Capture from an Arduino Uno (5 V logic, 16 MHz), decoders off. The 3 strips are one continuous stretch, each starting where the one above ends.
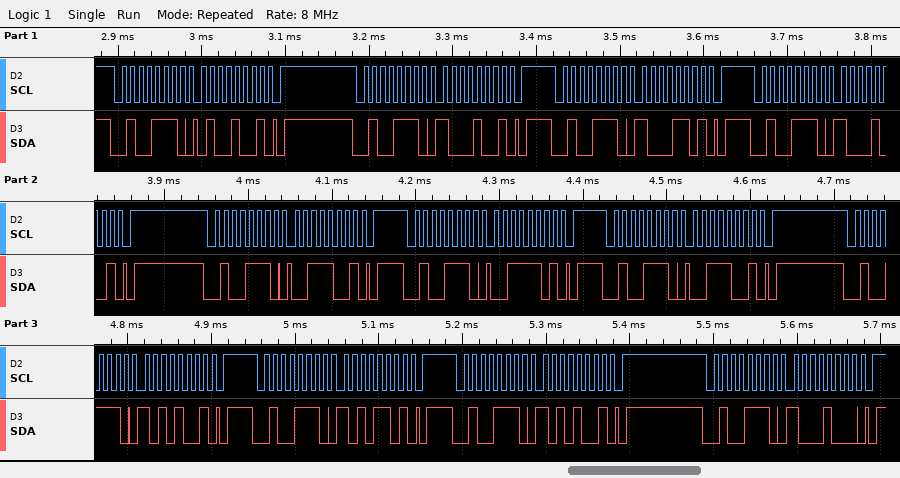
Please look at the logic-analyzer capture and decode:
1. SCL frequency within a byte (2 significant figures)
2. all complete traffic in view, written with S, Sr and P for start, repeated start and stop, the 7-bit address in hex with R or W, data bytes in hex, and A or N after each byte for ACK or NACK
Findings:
100 kHz
S 27W A 49 A P S 27W A 89 A P S 27W A 8D A P S 27W A 89 A P S 27W A 39 A P S 27W A 3D A P S 27W A 39 A P S 27W A A9 A P S 27W A AD A P S 27W A A9 A P S 27W A 88 A P
